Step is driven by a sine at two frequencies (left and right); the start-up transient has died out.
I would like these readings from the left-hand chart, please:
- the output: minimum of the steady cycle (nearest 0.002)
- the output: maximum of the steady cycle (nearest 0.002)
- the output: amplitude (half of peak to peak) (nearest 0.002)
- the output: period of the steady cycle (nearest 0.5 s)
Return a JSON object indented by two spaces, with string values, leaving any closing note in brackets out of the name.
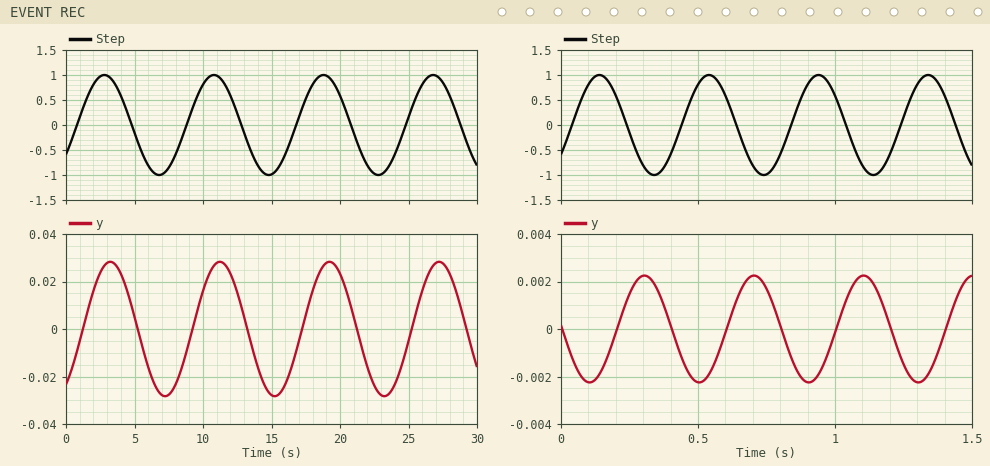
{
  "the output: minimum of the steady cycle": "-0.028",
  "the output: maximum of the steady cycle": "0.028",
  "the output: amplitude (half of peak to peak)": "0.028",
  "the output: period of the steady cycle": "8.0 s"
}
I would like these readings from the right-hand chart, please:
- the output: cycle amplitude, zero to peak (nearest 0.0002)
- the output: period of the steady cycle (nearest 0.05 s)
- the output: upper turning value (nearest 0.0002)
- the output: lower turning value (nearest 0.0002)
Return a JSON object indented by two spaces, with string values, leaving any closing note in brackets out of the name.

{
  "the output: cycle amplitude, zero to peak": "0.0022",
  "the output: period of the steady cycle": "0.40 s",
  "the output: upper turning value": "0.0022",
  "the output: lower turning value": "-0.0022"
}
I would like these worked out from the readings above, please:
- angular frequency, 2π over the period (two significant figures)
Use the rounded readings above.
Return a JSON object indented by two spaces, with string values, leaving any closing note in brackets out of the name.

{
  "angular frequency, 2π over the period": "16 rad/s"
}
